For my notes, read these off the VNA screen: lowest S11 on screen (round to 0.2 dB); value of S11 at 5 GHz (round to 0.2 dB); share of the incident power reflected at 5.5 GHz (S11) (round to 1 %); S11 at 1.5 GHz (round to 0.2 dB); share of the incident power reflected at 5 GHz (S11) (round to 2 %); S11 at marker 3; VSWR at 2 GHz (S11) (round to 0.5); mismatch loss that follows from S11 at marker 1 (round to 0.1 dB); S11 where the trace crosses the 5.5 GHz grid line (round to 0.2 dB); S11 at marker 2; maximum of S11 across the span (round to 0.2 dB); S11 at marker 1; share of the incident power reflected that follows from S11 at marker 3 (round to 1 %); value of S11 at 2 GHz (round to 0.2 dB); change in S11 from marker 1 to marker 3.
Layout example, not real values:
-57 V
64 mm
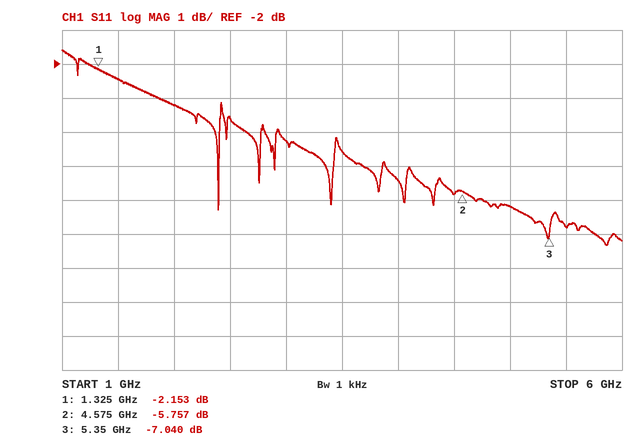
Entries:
-7.4 dB
-6.2 dB
21 %
-2.4 dB
24 %
-7.040 dB
5.5
4.1 dB
-6.8 dB
-5.757 dB
-1.6 dB
-2.153 dB
20 %
-3.2 dB
-4.887 dB
